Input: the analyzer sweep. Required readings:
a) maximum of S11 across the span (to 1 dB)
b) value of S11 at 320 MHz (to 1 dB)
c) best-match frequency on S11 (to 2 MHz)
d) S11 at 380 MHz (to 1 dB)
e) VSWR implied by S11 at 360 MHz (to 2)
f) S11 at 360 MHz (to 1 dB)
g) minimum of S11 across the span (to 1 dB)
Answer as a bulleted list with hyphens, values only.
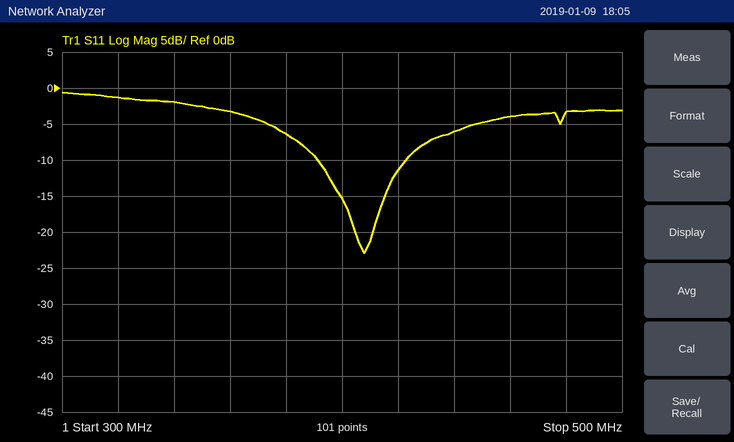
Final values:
- -1 dB
- -1 dB
- 408 MHz
- -6 dB
- 6
- -3 dB
- -23 dB
